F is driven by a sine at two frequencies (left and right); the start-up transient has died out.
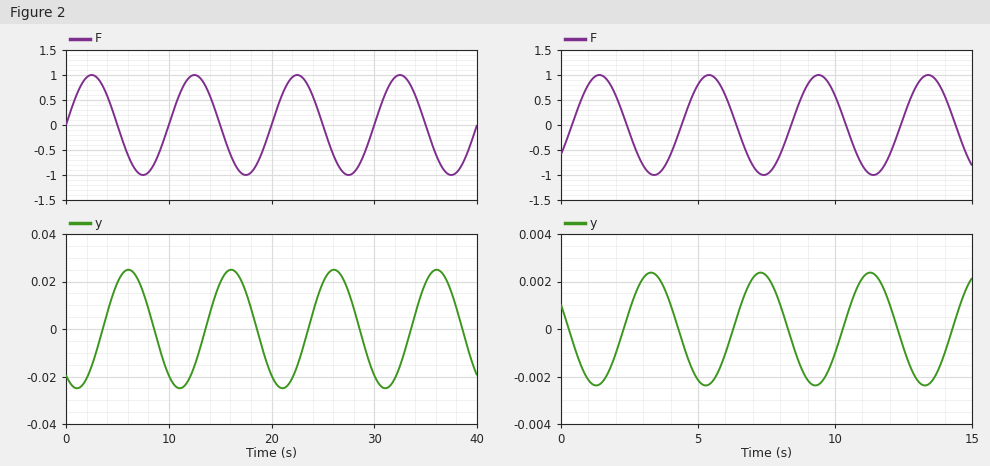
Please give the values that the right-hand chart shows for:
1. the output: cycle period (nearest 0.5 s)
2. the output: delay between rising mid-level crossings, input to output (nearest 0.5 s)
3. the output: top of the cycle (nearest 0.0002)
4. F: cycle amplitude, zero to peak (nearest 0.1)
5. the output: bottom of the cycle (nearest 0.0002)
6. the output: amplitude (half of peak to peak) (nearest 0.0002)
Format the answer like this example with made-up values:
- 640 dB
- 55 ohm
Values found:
- 4.0 s
- 2.0 s
- 0.0024
- 1.0
- -0.0024
- 0.0024
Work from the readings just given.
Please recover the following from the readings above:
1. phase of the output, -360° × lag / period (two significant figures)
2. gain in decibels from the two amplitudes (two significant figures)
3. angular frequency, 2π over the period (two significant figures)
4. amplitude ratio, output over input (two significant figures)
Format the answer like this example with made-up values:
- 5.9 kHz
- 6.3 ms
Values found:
- -180°
- -52 dB
- 1.6 rad/s
- 0.0024
